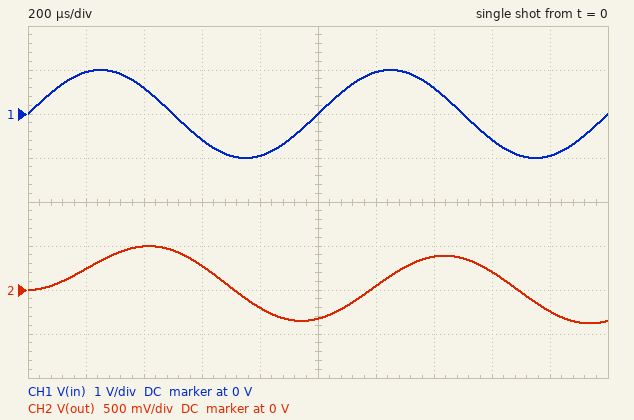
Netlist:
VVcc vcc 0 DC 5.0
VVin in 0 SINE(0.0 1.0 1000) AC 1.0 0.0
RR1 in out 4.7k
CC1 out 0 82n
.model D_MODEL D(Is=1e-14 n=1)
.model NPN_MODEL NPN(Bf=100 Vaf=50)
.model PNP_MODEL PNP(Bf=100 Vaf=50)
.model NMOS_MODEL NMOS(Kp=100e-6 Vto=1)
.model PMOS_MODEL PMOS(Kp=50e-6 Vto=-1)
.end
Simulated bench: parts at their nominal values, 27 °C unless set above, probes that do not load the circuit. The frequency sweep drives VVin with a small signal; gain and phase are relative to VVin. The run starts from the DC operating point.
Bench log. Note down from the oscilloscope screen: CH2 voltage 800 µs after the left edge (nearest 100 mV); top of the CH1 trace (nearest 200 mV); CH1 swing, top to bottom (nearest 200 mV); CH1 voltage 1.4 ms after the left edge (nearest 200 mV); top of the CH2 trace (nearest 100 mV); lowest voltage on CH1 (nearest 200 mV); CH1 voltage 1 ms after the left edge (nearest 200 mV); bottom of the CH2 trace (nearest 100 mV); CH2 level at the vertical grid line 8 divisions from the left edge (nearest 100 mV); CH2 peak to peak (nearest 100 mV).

-200 mV
1.0 V
2.0 V
600 mV
500 mV
-1.0 V
0 V
-400 mV
200 mV
900 mV
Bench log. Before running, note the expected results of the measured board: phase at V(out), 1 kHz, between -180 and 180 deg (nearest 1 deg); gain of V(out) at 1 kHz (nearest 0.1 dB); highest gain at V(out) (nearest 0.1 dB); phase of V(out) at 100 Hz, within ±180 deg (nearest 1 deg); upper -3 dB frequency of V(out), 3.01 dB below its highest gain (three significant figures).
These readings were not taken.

-68 deg
-8.4 dB
0 dB
-14 deg
413 Hz
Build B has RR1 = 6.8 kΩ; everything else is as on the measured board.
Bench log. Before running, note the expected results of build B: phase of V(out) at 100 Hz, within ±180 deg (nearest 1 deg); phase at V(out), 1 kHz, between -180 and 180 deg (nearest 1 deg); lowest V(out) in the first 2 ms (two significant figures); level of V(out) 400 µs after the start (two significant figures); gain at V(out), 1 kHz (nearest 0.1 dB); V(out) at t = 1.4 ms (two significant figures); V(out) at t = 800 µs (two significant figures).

-19 deg
-74 deg
-270 mV
390 mV
-11.2 dB
280 mV
-90 mV
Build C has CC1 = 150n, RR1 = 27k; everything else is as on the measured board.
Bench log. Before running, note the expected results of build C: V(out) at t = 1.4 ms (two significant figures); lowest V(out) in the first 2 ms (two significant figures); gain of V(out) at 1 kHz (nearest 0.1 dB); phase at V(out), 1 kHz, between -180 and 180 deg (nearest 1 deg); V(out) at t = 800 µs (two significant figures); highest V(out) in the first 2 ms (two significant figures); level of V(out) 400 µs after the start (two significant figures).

60 mV
-15 mV
-28.1 dB
-88 deg
19 mV
74 mV
68 mV
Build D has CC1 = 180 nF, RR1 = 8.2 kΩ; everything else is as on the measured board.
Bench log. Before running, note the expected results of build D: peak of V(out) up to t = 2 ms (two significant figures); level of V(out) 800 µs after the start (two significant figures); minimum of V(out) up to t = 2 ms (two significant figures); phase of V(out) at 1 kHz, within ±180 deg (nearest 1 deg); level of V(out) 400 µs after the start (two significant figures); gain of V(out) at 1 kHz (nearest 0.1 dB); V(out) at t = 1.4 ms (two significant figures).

180 mV
18 mV
-79 mV
-84 deg
170 mV
-19.4 dB
130 mV
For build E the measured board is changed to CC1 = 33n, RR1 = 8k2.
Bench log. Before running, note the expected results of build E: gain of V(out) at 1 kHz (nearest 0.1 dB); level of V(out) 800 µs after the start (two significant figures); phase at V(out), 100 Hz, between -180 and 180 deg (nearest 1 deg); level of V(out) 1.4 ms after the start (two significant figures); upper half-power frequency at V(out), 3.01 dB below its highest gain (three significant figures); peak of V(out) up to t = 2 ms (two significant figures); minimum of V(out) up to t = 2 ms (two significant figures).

-5.9 dB
-360 mV
-10 deg
510 mV
588 Hz
600 mV
-510 mV
